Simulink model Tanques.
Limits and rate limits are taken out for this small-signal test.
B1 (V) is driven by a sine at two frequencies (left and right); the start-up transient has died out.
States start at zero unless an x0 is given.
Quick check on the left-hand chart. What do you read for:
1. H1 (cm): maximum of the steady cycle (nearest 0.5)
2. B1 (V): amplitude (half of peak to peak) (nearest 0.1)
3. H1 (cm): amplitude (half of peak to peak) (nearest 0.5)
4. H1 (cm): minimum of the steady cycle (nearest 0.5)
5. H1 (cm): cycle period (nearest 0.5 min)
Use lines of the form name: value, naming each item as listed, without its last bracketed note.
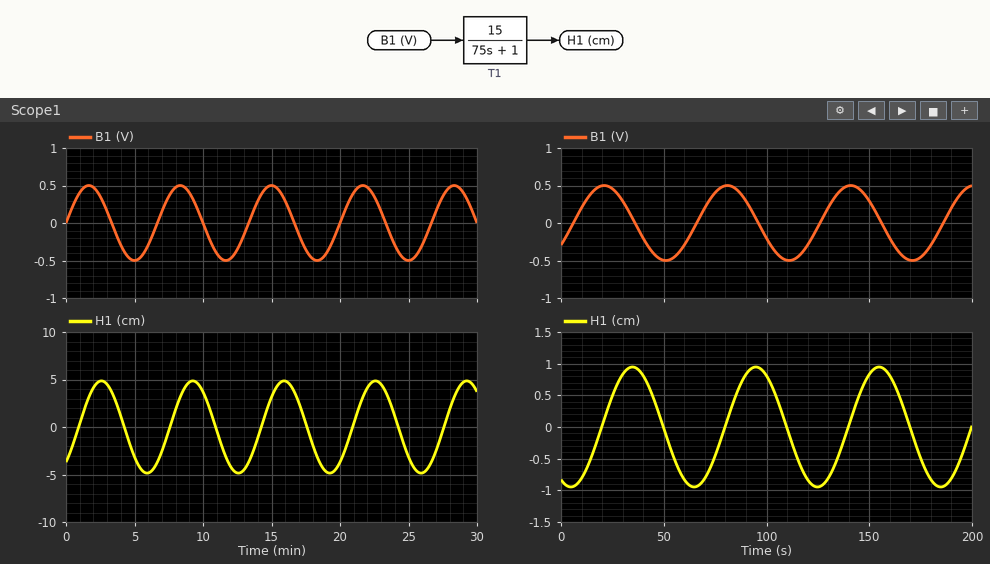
H1 (cm): maximum of the steady cycle: 5.0
B1 (V): amplitude (half of peak to peak): 0.5
H1 (cm): amplitude (half of peak to peak): 5.0
H1 (cm): minimum of the steady cycle: -5.0
H1 (cm): cycle period: 6.5 min
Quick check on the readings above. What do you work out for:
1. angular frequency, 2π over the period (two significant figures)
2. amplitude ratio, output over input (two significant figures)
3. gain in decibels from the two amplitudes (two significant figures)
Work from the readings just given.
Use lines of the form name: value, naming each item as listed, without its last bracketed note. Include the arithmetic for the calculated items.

angular frequency, 2π over the period: 2π / 6.5 = 0.97 rad/min
amplitude ratio, output over input: 5 / 0.5 = 10
gain in decibels from the two amplitudes: 20 log10(5 / 0.5) = 20 dB
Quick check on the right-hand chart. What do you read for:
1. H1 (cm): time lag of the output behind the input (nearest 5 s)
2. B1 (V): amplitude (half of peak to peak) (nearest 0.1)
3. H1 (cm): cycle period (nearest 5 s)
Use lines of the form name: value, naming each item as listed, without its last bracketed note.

H1 (cm): time lag of the output behind the input: 15 s
B1 (V): amplitude (half of peak to peak): 0.5
H1 (cm): cycle period: 60 s
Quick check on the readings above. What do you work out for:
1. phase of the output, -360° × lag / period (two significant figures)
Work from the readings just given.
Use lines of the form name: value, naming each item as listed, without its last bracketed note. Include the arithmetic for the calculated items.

phase of the output, -360° × lag / period: -360 × 15 / 60 = -90°
